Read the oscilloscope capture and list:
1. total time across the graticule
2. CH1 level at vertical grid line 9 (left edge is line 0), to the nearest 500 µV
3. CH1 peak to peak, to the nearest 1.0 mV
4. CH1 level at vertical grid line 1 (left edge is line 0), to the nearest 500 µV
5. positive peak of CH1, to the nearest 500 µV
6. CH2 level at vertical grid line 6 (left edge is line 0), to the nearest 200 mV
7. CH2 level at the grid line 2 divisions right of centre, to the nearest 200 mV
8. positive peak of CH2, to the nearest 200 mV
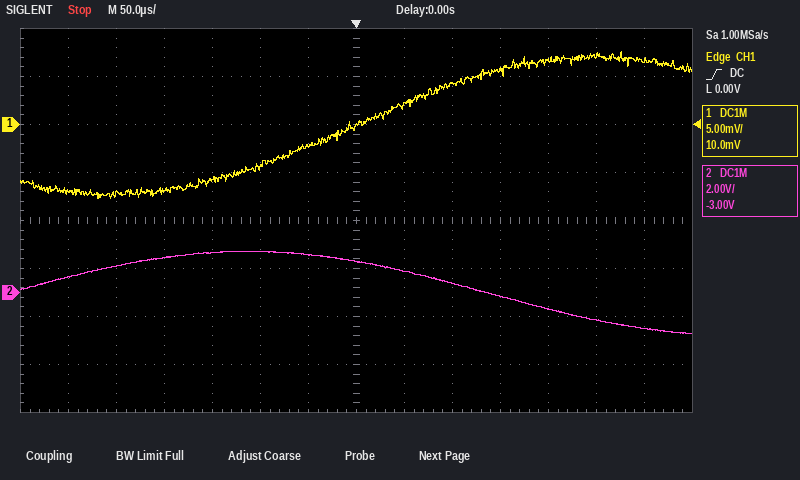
700 µs
4.5 mV
15.0 mV
-7.0 mV
7.5 mV
1.6 V
400 mV
1.8 V
